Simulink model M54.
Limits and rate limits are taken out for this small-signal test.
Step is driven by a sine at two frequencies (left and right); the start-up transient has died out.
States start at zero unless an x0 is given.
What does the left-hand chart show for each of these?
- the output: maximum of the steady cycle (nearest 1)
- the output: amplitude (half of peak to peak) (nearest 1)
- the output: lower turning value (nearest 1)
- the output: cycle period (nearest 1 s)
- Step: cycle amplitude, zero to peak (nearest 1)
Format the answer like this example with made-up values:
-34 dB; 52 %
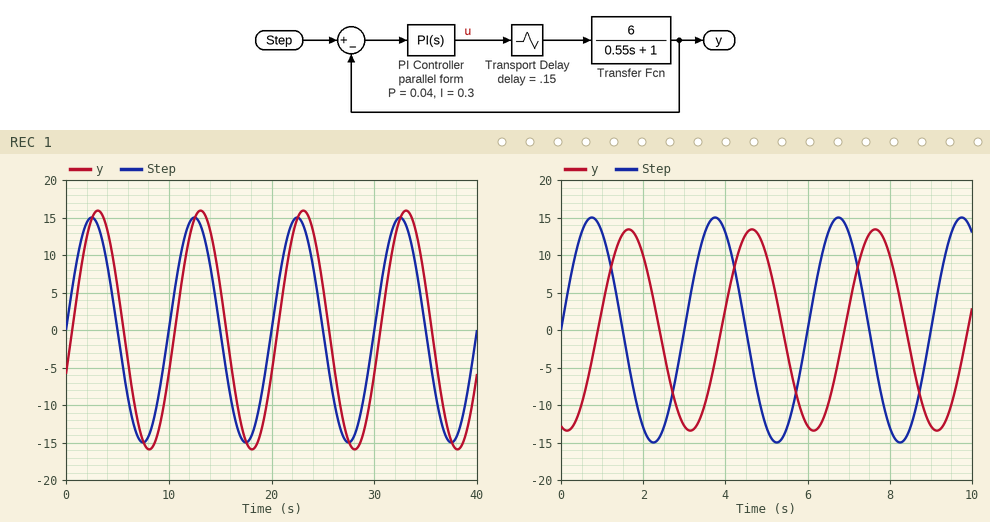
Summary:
16; 16; -16; 10 s; 15
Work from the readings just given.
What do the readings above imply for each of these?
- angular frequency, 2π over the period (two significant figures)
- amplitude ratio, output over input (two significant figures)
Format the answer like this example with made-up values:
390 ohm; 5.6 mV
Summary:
0.63 rad/s; 1.1
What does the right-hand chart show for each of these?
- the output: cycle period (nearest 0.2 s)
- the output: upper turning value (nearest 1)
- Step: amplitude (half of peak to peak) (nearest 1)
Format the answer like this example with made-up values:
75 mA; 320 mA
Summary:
3.0 s; 13; 15
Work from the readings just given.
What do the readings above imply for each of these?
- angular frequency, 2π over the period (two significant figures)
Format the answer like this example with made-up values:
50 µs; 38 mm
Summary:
2.1 rad/s
